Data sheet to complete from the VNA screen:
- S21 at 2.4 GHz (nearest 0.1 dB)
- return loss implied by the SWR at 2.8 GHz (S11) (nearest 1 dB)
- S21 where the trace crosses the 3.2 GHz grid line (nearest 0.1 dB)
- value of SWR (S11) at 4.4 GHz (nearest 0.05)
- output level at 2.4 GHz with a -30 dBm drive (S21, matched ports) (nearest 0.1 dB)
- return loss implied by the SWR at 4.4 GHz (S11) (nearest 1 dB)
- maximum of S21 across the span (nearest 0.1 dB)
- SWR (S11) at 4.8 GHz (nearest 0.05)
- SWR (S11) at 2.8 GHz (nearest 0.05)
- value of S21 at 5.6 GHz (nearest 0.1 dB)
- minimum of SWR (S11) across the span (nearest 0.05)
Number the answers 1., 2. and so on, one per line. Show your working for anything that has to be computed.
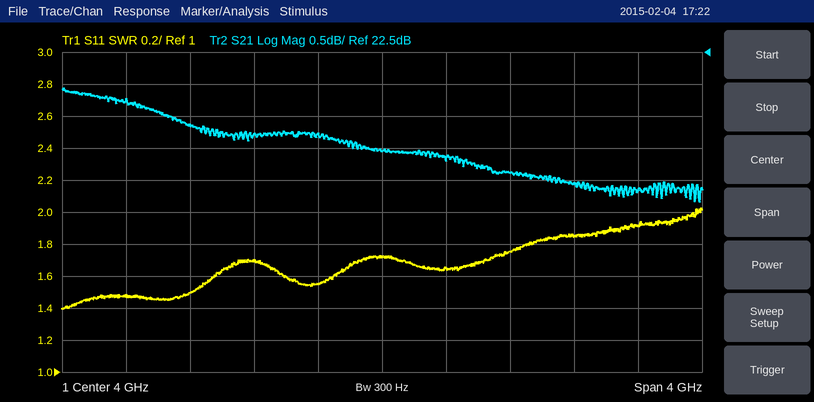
1. 21.7 dB
2. −20 log10((1.5 − 1)/(1.5 + 1)) ≈ 14 dB
3. 21.2 dB
4. 1.65
5. -30 dBm + (21.7 dB) = -8.3 dBm
6. −20 log10((1.65 − 1)/(1.65 + 1)) ≈ 12 dB
7. 21.9 dB
8. 1.75
9. 1.50
10. 20.3 dB
11. 1.40
